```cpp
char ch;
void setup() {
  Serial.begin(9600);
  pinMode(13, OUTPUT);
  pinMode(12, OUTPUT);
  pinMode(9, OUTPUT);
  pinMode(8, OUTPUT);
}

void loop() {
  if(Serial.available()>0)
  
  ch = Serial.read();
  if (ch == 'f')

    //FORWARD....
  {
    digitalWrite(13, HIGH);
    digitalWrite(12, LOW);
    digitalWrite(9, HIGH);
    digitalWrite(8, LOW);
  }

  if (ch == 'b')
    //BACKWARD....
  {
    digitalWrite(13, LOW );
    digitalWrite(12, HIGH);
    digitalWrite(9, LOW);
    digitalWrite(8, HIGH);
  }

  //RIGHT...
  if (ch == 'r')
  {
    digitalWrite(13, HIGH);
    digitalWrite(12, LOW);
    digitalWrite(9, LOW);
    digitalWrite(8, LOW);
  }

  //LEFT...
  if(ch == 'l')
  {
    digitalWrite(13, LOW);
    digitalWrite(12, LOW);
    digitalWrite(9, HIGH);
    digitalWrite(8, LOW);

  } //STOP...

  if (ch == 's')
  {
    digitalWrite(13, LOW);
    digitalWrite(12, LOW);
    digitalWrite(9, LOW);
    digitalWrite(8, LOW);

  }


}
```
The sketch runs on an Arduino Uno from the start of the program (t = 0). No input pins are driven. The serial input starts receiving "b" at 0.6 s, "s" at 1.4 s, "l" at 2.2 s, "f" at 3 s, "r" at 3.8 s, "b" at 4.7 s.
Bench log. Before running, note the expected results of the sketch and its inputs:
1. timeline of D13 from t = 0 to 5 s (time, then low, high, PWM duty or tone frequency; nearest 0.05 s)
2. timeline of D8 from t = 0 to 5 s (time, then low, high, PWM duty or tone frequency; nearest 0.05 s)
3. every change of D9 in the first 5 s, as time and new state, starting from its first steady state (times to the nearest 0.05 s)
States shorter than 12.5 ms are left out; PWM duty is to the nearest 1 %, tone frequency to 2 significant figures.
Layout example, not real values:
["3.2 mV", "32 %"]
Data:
["0 s low; 3 s high; 4.7 s low", "0 s low; 0.6 s high; 1.4 s low; 4.7 s high", "0 s low; 2.2 s high; 3.8 s low"]
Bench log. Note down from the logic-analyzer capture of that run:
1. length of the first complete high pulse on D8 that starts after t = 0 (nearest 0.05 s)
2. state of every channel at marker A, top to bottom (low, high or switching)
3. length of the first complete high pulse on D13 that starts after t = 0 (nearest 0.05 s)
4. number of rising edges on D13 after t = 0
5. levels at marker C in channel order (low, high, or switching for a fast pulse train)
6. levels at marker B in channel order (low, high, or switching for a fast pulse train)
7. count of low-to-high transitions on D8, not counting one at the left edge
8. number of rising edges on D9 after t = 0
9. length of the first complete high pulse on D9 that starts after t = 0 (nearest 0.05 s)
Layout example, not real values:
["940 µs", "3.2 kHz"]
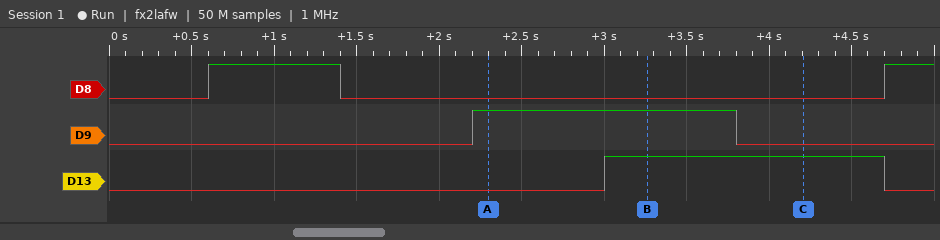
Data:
["0.80 s", "D8 low, D9 high, D13 low", "1.70 s", "1", "D8 low, D9 low, D13 high", "D8 low, D9 high, D13 high", "2", "1", "1.60 s"]
